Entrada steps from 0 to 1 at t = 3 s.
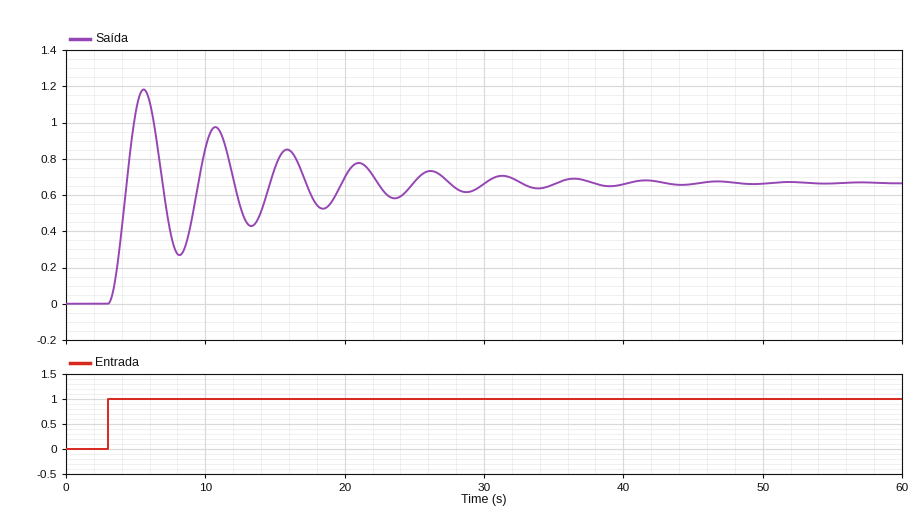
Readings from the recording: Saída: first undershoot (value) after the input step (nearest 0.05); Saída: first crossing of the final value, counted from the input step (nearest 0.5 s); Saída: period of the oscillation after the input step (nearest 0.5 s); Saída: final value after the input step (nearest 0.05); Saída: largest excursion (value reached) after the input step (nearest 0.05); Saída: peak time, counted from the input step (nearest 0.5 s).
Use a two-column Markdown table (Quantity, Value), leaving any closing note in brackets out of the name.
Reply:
| Quantity | Value |
|---|---|
| Saída: first undershoot (value) after the input step | 0.25 |
| Saída: first crossing of the final value, counted from the input step | 1.5 s |
| Saída: period of the oscillation after the input step | 5.0 s |
| Saída: final value after the input step | 0.65 |
| Saída: largest excursion (value reached) after the input step | 1.20 |
| Saída: peak time, counted from the input step | 2.5 s |
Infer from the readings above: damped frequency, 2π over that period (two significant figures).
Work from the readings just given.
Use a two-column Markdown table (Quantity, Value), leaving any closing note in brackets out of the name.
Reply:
| Quantity | Value |
|---|---|
| damped frequency, 2π over that period | 1.3 rad/s |
